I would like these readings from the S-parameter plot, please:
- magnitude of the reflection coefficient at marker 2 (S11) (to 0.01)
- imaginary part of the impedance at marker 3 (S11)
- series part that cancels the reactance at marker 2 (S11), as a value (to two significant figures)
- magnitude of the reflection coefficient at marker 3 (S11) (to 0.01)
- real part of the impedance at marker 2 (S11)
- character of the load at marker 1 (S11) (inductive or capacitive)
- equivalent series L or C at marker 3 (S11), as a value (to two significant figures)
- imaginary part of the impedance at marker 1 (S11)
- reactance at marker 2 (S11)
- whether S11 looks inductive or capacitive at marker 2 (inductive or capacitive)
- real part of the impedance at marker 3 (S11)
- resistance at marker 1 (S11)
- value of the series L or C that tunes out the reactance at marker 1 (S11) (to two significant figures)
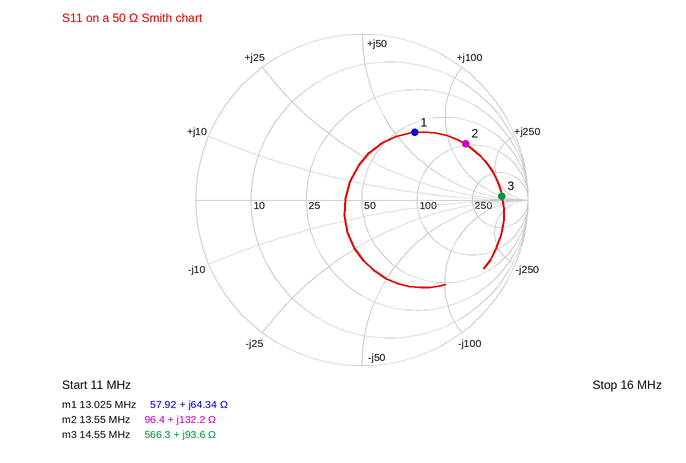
0.71
+93.6 Ω
89 pF
0.84
96.4 Ω
inductive
1.0 µH
+64.34 Ω
+132.2 Ω
inductive
566.3 Ω
57.92 Ω
190 pF
